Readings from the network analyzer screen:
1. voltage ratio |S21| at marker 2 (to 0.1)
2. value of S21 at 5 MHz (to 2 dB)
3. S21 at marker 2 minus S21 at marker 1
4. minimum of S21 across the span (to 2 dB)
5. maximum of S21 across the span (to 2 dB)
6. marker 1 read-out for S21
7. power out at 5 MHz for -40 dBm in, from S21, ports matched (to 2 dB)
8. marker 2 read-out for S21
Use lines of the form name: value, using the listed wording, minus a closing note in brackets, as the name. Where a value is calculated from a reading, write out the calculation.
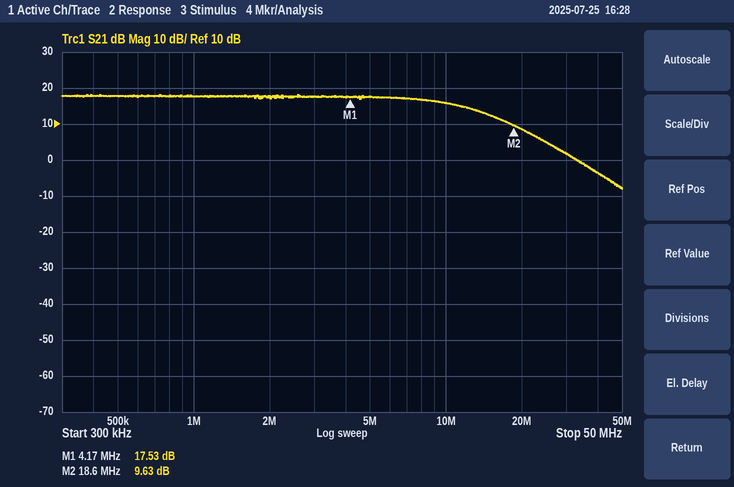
voltage ratio |S21| at marker 2: 10^(9.63/20) ≈ 3.0
value of S21 at 5 MHz: 18 dB
S21 at marker 2 minus S21 at marker 1: 9.63 − (17.53) = -7.90 dB
minimum of S21 across the span: -8 dB
maximum of S21 across the span: 18 dB
marker 1 read-out for S21: 17.53 dB
power out at 5 MHz for -40 dBm in, from S21, ports matched: -40 dBm + (18 dB) = -22 dBm
marker 2 read-out for S21: 9.63 dB
